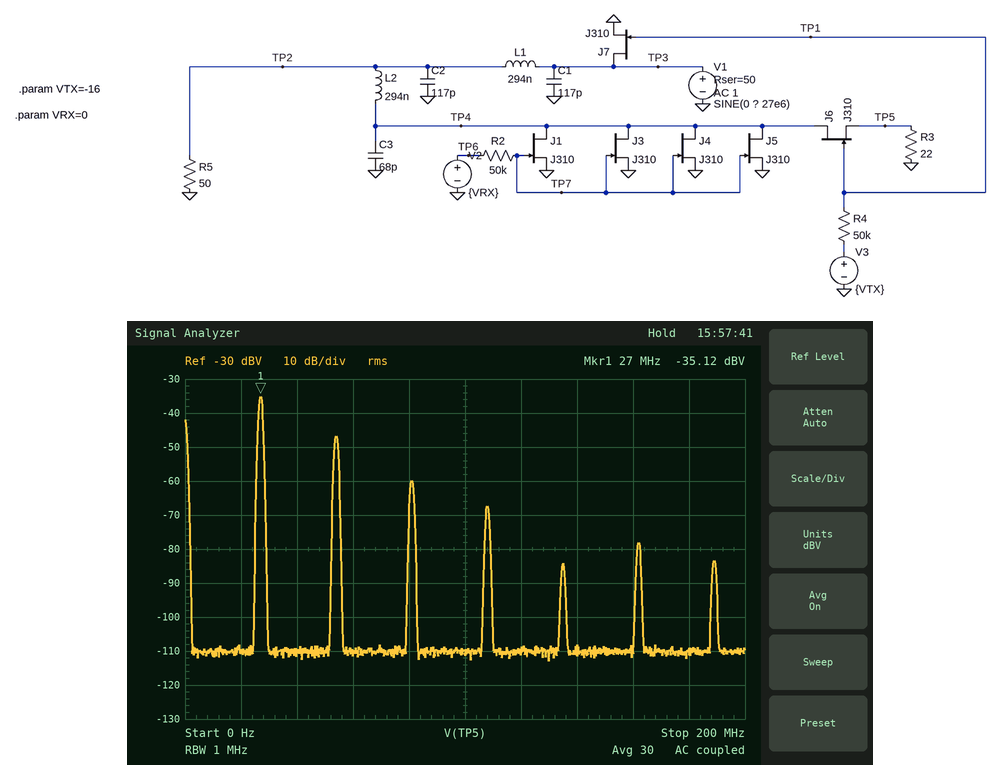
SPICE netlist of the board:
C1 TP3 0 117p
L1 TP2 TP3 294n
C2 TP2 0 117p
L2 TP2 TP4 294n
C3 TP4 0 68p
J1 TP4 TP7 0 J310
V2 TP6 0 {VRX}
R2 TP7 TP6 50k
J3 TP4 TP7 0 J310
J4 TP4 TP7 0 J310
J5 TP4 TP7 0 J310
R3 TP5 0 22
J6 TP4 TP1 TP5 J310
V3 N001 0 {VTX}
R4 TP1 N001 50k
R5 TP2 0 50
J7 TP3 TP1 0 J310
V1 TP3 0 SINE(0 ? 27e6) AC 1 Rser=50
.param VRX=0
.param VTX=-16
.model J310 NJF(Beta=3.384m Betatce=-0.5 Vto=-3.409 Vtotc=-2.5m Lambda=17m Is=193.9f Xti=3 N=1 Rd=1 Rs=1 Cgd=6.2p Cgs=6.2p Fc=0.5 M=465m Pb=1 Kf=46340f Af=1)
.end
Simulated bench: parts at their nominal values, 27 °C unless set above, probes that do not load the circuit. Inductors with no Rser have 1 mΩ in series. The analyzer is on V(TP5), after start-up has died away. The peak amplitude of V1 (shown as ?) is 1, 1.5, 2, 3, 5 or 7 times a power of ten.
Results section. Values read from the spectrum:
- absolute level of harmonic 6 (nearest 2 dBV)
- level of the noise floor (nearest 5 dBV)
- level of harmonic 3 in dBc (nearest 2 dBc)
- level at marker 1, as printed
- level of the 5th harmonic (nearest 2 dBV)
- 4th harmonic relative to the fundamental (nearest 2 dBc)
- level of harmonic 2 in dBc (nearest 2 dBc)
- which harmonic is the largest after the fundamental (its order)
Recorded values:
-78 dBV
-110 dBV
-24 dBc
-35.12 dBV
-84 dBV
-32 dBc
-12 dBc
2
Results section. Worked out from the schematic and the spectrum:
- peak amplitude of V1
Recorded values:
30 V
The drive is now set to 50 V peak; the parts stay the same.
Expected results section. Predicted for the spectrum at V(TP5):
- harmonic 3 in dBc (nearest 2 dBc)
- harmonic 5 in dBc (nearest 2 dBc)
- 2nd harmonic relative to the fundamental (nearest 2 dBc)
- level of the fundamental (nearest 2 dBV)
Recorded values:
-12 dBc
-6 dBc
4 dBc
-38 dBV
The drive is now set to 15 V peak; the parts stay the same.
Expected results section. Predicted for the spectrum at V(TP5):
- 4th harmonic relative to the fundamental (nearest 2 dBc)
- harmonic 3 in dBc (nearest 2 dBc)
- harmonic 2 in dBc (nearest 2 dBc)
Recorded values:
-58 dBc
-40 dBc
-20 dBc
